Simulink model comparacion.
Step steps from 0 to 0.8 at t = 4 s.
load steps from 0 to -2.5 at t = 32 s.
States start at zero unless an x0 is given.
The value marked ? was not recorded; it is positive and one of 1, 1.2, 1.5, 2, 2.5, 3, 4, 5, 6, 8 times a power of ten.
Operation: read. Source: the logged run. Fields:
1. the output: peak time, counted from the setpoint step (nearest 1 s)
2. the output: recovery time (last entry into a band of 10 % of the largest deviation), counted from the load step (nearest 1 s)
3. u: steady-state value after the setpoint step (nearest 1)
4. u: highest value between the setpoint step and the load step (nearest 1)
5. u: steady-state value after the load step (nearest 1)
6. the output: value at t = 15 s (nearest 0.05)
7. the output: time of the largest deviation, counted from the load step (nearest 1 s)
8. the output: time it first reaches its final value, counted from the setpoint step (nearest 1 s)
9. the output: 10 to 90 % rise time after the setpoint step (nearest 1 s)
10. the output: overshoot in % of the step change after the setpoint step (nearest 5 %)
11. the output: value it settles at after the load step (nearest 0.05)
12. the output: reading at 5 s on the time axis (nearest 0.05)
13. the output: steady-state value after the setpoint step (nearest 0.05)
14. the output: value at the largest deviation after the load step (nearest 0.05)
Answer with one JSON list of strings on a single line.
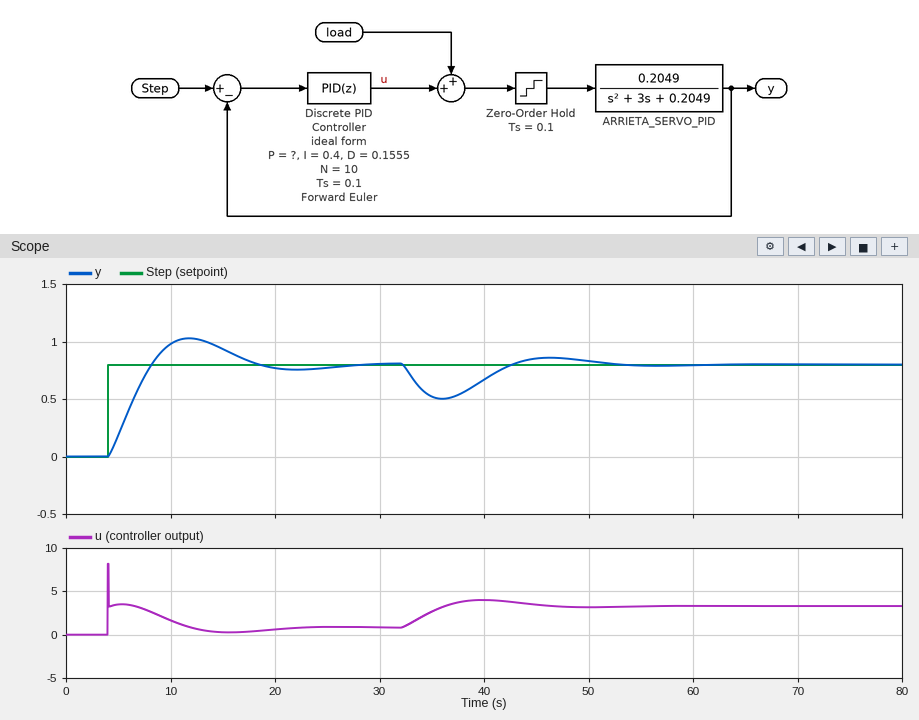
["8 s", "18 s", "1", "8", "3", "0.95", "4 s", "4 s", "3 s", "30 %", "0.80", "0.20", "0.80", "0.50"]
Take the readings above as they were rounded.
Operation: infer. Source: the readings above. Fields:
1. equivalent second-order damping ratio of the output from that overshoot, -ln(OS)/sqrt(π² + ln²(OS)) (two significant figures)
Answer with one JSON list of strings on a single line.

["0.36"]
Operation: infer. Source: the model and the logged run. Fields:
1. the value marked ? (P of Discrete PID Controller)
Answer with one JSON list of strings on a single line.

["4"]
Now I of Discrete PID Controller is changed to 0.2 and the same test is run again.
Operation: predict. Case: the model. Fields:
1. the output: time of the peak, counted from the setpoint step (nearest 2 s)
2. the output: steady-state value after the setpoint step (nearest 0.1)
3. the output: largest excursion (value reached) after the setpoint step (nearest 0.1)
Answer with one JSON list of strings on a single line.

["10 s", "0.8", "0.9"]
